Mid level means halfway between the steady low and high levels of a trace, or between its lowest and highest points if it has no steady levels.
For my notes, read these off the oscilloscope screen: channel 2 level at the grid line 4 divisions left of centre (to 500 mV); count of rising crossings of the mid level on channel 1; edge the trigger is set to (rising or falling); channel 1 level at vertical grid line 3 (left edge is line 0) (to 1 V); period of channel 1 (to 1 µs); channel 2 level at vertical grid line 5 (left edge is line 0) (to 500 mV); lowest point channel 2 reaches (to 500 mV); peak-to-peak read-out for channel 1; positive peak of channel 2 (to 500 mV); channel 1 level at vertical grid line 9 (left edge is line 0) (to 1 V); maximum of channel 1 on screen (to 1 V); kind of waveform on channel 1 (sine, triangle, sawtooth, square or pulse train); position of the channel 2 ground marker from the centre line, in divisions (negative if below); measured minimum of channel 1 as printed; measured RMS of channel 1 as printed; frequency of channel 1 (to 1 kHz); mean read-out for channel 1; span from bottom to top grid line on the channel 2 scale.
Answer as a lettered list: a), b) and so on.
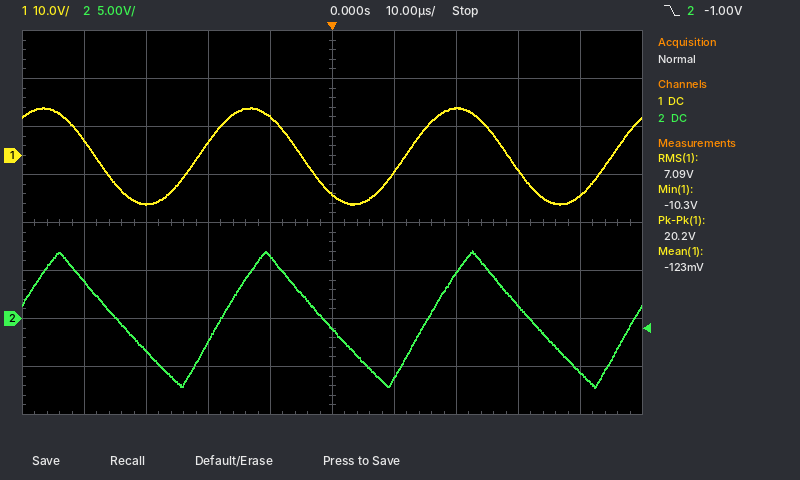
a) 4.0 V
b) 3
c) falling
d) 3 V
e) 33 µs
f) -1.0 V
g) -7.0 V
h) 20.2 V
i) 7.0 V
j) -8 V
k) 10 V
l) sine
m) -2.0 div
n) -10.3 V
o) 7.09 V
p) 30 kHz
q) -123 mV
r) 40 V
